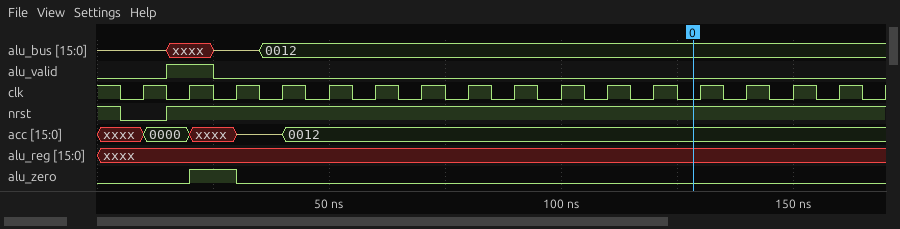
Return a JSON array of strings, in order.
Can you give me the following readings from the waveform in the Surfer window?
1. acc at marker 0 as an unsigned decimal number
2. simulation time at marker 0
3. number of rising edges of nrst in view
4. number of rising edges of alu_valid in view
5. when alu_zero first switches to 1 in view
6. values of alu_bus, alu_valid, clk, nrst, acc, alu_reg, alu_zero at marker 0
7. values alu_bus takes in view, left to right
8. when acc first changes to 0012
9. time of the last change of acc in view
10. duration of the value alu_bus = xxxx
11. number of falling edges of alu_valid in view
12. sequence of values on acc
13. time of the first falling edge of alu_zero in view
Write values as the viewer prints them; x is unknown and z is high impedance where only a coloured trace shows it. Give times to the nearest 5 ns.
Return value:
["18", "130 ns", "1", "1", "20 ns", "alu_bus=0012, alu_valid=0, clk=0, nrst=1, acc=0012, alu_reg=xxxx, alu_zero=0", "z, xxxx, z, 0012", "40 ns", "40 ns", "10 ns", "1", "xxxx, 0000, xxxx, z, 0012", "30 ns"]
